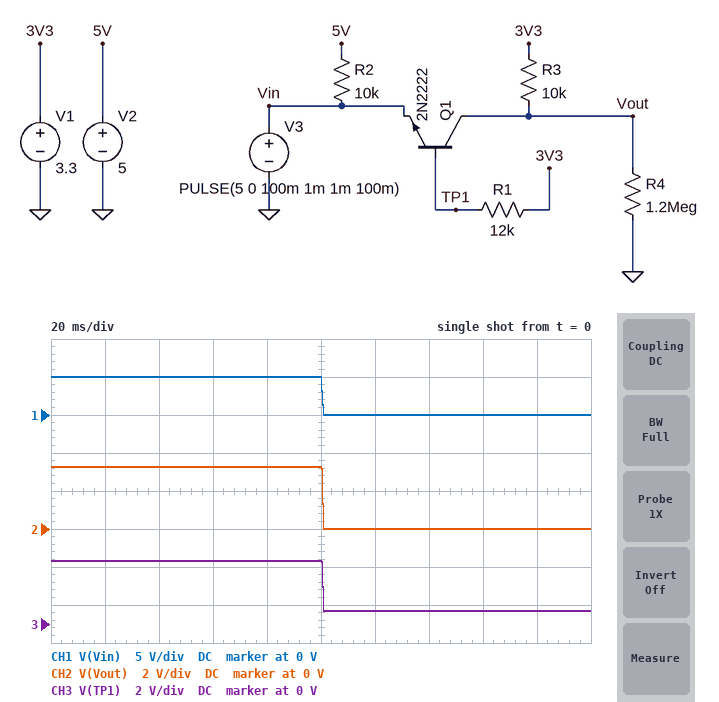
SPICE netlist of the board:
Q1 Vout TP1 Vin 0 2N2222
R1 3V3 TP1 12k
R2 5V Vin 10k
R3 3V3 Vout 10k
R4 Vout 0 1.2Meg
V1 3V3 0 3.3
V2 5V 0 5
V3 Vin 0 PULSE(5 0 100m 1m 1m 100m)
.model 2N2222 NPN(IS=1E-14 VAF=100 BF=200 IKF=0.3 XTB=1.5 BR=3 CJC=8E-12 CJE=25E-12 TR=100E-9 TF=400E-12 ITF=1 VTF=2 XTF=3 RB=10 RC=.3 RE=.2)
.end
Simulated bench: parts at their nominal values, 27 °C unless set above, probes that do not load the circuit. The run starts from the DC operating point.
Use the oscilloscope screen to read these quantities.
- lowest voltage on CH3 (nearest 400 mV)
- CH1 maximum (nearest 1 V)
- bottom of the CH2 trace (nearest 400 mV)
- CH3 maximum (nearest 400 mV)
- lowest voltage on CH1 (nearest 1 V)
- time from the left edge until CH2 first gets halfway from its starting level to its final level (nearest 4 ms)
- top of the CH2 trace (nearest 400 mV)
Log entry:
800 mV
5 V
0 V
3.2 V
0 V
100 ms
3.2 V
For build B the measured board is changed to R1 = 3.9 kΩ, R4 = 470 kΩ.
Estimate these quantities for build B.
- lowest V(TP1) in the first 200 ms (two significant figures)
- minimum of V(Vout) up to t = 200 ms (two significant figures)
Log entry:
690 mV
11 mV
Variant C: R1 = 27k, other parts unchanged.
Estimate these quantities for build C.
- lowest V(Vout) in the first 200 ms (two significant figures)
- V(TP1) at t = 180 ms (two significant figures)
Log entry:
24 mV
650 mV
